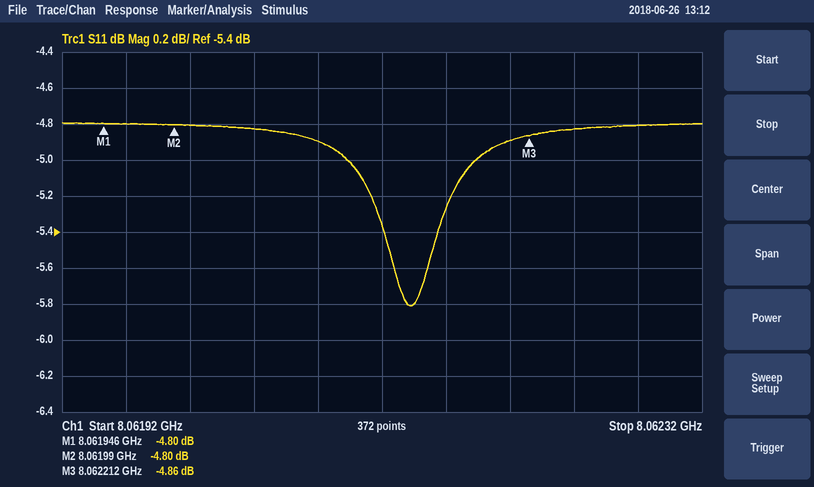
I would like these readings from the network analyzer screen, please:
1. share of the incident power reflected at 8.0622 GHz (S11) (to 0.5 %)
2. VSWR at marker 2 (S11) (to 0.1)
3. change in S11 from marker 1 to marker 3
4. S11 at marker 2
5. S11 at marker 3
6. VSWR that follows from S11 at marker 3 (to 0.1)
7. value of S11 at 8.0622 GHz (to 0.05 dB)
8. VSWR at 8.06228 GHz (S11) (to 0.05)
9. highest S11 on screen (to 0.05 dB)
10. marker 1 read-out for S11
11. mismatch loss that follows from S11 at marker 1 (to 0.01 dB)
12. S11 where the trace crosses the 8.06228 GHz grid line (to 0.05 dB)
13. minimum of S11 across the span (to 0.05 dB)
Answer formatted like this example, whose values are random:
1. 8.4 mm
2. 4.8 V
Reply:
1. 32.5 %
2. 3.7
3. -0.06 dB
4. -4.80 dB
5. -4.86 dB
6. 3.7
7. -4.90 dB
8. 3.70
9. -4.80 dB
10. -4.80 dB
11. 1.75 dB
12. -4.80 dB
13. -5.80 dB
